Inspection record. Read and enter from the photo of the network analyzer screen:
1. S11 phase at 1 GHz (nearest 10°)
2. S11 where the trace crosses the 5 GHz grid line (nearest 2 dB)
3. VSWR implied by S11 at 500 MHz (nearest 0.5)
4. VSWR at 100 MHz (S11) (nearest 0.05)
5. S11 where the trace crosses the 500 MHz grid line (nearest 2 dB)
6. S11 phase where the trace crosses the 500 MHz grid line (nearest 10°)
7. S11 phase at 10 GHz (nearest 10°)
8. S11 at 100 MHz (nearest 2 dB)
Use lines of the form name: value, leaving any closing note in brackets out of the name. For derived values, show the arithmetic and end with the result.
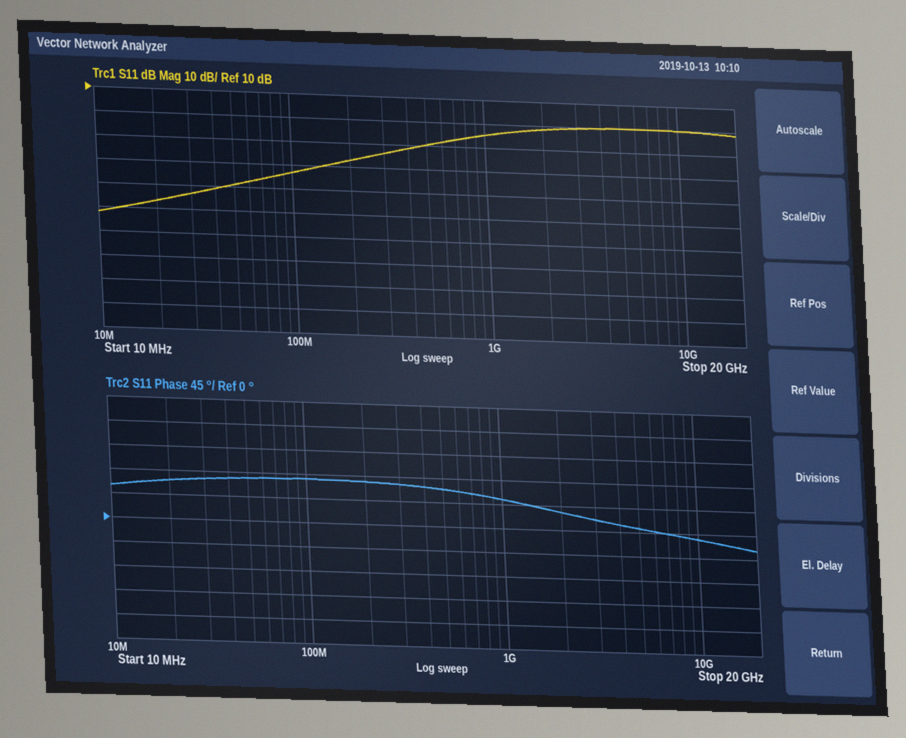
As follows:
S11 phase at 1 GHz: 50°
S11 where the trace crosses the 5 GHz grid line: 0 dB
VSWR implied by S11 at 500 MHz: |Γ| = 10^(-10/20) = 0.3162; VSWR = (1 + 0.3162)/(1 − 0.3162) ≈ 1.92, so 2.0 to the nearest 0.5
VSWR at 100 MHz (S11): |Γ| = 10^(-24/20) = 0.0631; VSWR = (1 + 0.0631)/(1 − 0.0631) ≈ 1.13, so 1.15 to the nearest 0.05
S11 where the trace crosses the 500 MHz grid line: -10 dB
S11 phase where the trace crosses the 500 MHz grid line: 70°
S11 phase at 10 GHz: -10°
S11 at 100 MHz: -24 dB
